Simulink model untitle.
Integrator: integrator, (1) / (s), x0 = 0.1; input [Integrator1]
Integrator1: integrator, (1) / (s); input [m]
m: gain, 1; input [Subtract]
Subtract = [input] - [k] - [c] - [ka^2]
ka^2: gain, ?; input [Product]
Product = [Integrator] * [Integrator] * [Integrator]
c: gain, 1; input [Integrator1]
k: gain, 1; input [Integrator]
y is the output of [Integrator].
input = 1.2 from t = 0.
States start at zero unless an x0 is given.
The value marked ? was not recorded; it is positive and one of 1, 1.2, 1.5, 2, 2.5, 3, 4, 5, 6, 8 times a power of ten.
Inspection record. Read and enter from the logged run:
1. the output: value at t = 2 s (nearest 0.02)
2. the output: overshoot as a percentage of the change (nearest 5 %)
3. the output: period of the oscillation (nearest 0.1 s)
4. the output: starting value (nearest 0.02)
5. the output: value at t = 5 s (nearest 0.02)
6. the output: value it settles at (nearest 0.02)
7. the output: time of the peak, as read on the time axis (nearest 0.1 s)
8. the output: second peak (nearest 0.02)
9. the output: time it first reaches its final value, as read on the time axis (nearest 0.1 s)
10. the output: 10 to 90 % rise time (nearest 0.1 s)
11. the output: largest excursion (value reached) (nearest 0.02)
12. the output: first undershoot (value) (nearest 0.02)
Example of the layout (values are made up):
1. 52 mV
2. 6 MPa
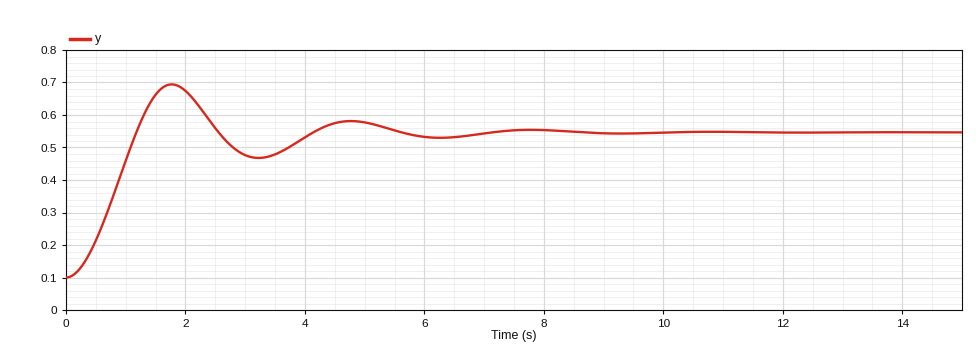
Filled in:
1. 0.68
2. 35 %
3. 3.0 s
4. 0.10
5. 0.58
6. 0.54
7. 1.8 s
8. 0.58
9. 1.2 s
10. 0.8 s
11. 0.70
12. 0.46
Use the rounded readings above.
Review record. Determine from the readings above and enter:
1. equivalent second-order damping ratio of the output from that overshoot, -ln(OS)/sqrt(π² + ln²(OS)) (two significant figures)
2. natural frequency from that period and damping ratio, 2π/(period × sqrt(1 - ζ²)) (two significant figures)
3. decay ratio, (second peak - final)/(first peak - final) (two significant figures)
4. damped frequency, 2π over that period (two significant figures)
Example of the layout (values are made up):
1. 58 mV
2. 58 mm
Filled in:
1. 0.32
2. 2.2 rad/s
3. 0.25
4. 2.1 rad/s
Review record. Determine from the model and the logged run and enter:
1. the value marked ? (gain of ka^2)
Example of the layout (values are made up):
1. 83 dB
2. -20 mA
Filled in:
1. 4
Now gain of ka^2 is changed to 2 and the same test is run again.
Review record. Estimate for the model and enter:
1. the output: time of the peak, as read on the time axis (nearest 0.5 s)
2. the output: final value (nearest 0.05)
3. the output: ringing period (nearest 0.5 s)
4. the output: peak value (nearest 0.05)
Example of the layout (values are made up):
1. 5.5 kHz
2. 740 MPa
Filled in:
1. 2.0 s
2. 0.65
3. 3.5 s
4. 0.80
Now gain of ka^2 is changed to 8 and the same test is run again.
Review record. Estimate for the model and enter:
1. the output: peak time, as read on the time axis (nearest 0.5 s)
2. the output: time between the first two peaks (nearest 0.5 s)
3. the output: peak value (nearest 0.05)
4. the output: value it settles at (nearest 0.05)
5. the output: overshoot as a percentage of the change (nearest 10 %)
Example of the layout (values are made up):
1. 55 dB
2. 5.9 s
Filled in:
1. 1.5 s
2. 2.5 s
3. 0.60
4. 0.45
5. 40 %
